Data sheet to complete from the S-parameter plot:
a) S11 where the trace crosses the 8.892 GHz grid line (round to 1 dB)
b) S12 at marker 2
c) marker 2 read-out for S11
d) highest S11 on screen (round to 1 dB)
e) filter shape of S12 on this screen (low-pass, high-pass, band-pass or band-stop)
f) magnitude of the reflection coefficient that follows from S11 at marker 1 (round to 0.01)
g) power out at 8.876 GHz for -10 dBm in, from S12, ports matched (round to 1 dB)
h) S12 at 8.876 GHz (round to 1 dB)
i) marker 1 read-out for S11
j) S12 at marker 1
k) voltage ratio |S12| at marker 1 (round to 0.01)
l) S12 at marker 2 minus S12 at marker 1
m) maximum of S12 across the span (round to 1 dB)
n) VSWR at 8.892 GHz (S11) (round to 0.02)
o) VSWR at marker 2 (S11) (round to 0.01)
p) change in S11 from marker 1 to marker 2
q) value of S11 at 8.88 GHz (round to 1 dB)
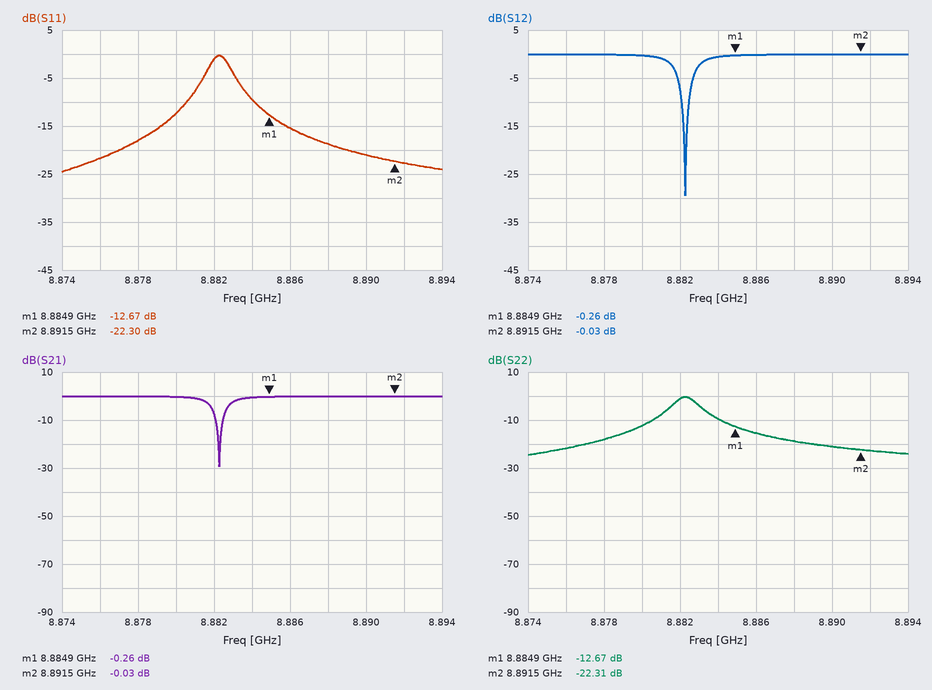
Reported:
-23 dB
-0.03 dB
-22.30 dB
0 dB
band-stop
0.23
-10 dBm
0 dB
-12.67 dB
-0.26 dB
0.97
0.23 dB
0 dB
1.16
1.17
-9.63 dB
-12 dB
